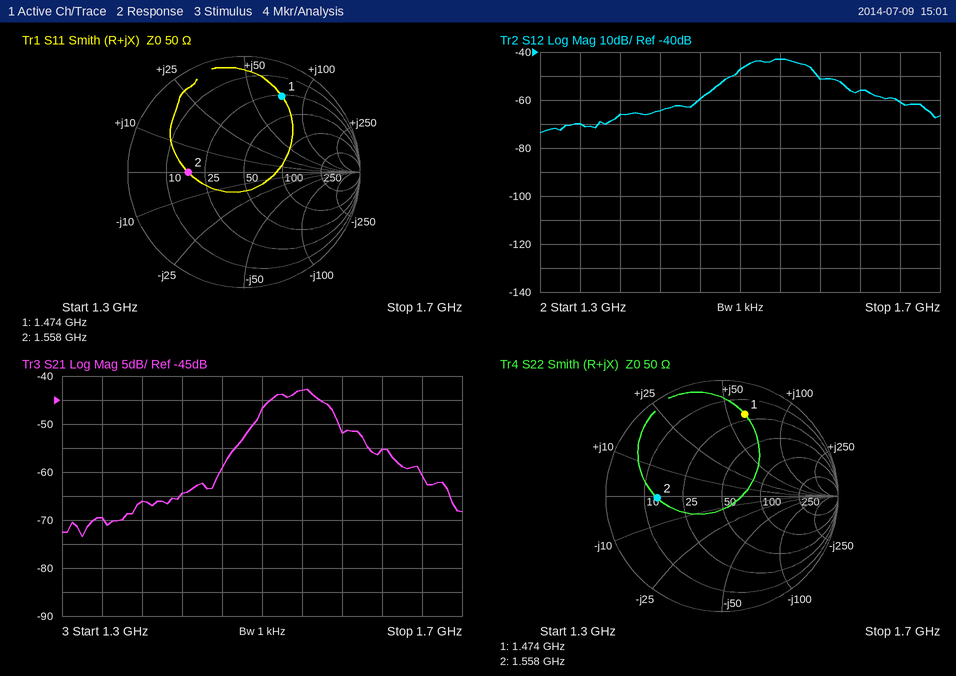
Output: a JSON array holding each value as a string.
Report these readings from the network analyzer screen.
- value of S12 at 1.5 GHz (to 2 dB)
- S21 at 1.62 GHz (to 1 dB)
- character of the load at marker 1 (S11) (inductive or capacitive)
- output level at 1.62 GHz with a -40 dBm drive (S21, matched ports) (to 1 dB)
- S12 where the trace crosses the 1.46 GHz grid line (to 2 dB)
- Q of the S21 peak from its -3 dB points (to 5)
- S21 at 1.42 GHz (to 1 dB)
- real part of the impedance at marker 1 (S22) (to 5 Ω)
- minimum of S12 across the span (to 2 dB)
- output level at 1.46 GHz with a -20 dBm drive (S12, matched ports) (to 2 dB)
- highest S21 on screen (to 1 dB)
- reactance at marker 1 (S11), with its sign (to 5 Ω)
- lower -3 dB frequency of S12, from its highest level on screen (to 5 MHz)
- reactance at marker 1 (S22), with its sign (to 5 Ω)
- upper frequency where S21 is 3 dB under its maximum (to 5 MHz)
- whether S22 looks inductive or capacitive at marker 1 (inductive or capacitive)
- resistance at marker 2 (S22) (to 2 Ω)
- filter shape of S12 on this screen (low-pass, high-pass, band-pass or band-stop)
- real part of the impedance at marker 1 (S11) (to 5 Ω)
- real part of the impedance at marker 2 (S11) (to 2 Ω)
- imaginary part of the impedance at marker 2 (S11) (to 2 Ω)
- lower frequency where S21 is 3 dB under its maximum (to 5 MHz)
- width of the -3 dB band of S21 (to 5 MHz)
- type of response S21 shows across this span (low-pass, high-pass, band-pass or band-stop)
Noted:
["-48 dB", "-55 dB", "inductive", "-95 dBm", "-60 dB", "25", "-64 dB", "20 Ω", "-74 dB", "-80 dBm", "-43 dB", "+75 Ω", "1.505 GHz", "+60 Ω", "1.565 GHz", "inductive", "14 Ω", "band-pass", "25 Ω", "18 Ω", "0 Ω", "1.505 GHz", "60 MHz", "band-pass"]
